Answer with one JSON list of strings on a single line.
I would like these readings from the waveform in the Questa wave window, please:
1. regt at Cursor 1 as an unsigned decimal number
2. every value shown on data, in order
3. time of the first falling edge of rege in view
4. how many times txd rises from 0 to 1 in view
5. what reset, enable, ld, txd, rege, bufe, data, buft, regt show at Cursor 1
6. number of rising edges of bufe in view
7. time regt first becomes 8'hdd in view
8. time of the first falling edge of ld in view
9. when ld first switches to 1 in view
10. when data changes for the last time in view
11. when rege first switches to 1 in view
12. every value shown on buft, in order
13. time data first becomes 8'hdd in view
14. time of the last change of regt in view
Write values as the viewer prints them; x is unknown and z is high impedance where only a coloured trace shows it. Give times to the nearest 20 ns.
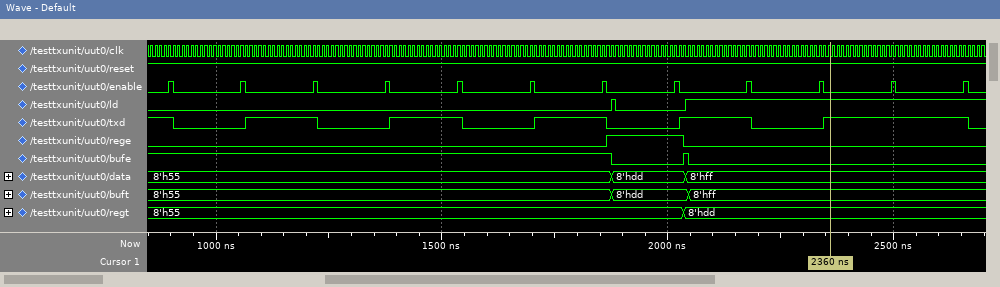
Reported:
["221", "8'h55, 8'hdd, 8'hff", "2040 ns", "5", "reset=1, enable=0, ld=1, txd=1, rege=0, bufe=0, data=8'hff, buft=8'hff, regt=8'hdd", "1", "2040 ns", "1880 ns", "1880 ns", "2040 ns", "1860 ns", "8'h55, 8'hdd, 8'hff", "1880 ns", "2040 ns"]
